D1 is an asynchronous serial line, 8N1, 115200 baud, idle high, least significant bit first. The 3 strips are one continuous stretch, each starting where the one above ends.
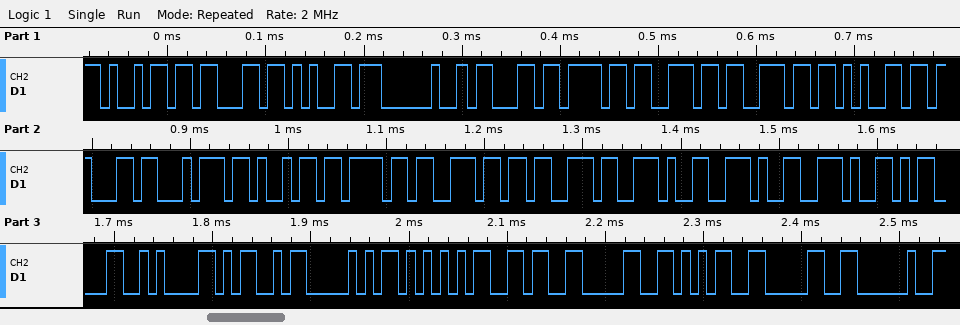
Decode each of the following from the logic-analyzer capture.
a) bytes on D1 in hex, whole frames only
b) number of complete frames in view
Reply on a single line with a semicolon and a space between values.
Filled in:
0x69 0x63 0x65 0x20 0x63 0x6F 0x6E 0x6E 0x65 0x63 0x74 0x69 0x6F 0x6E 0x73 0x2E 0x2E 0x2E 0x0D 0x0A 0x4D 0x50 0x55 0x36 0x30 0x35 0x30 0x20; 28
